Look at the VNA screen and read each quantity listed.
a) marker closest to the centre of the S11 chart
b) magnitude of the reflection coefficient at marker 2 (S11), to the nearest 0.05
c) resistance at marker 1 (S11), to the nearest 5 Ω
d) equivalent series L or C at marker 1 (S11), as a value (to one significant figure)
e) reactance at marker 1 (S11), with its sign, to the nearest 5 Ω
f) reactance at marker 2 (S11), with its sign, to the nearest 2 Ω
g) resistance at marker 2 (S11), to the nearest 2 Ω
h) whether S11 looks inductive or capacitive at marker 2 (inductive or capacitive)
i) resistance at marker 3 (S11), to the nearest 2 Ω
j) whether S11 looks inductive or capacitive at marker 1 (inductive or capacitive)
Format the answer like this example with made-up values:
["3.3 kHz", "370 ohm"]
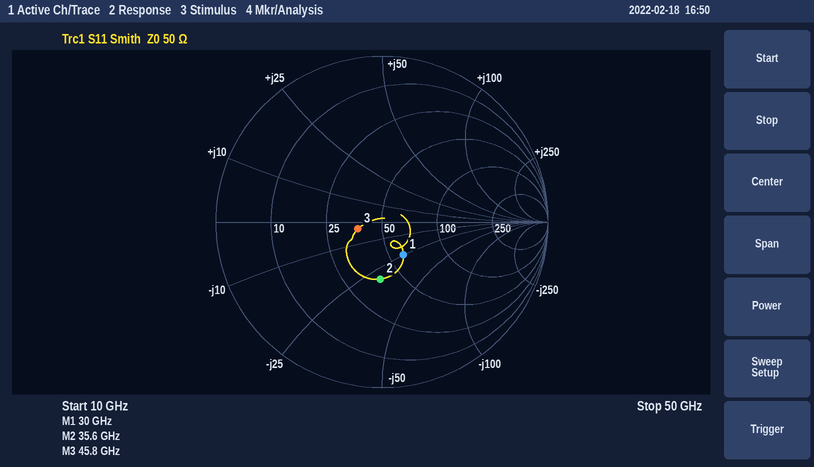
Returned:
["marker 3", "0.35", "60 Ω", "200 fF", "-25 Ω", "-30 Ω", "38 Ω", "capacitive", "38 Ω", "capacitive"]
